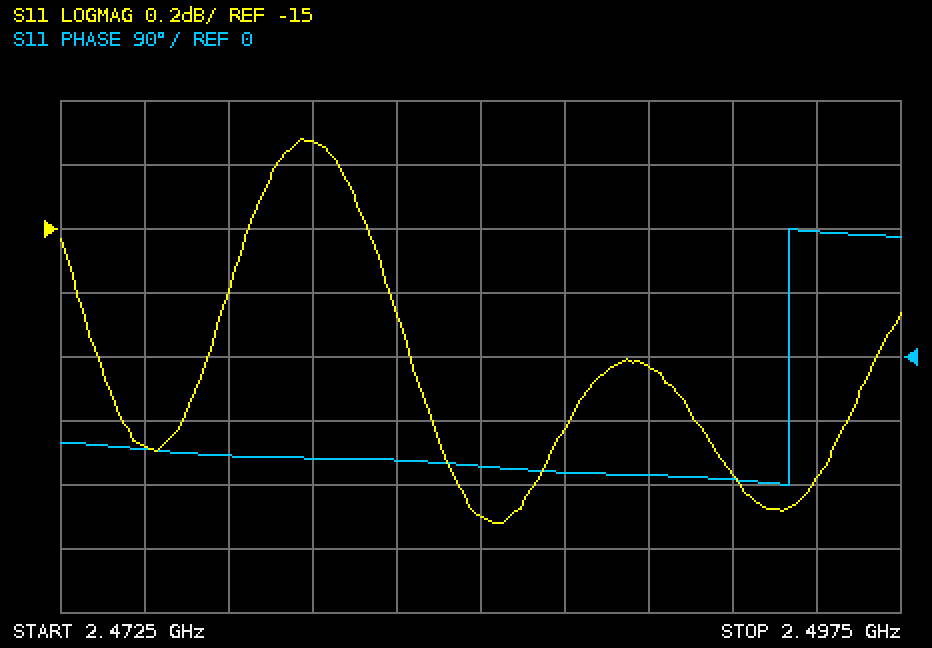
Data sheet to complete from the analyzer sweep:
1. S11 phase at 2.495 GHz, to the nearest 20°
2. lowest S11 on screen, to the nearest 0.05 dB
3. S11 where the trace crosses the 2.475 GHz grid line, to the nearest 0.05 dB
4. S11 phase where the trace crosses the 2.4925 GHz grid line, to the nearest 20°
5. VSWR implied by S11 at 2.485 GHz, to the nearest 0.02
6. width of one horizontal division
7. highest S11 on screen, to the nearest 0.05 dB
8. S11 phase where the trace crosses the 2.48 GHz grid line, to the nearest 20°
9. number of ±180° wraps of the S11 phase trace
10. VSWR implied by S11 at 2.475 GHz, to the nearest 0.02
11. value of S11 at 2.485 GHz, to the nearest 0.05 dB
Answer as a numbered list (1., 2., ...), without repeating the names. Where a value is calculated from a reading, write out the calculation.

1. 180°
2. -15.90 dB
3. -15.70 dB
4. -180°
5. |Γ| = 10^(-15.9/20) = 0.1603; VSWR = (1 + 0.1603)/(1 − 0.1603) ≈ 1.38
6. 2.5 MHz
7. -14.70 dB
8. -140°
9. 1
10. |Γ| = 10^(-15.7/20) = 0.1641; VSWR = (1 + 0.1641)/(1 − 0.1641) ≈ 1.39, so 1.40 to the nearest 0.02
11. -15.90 dB
